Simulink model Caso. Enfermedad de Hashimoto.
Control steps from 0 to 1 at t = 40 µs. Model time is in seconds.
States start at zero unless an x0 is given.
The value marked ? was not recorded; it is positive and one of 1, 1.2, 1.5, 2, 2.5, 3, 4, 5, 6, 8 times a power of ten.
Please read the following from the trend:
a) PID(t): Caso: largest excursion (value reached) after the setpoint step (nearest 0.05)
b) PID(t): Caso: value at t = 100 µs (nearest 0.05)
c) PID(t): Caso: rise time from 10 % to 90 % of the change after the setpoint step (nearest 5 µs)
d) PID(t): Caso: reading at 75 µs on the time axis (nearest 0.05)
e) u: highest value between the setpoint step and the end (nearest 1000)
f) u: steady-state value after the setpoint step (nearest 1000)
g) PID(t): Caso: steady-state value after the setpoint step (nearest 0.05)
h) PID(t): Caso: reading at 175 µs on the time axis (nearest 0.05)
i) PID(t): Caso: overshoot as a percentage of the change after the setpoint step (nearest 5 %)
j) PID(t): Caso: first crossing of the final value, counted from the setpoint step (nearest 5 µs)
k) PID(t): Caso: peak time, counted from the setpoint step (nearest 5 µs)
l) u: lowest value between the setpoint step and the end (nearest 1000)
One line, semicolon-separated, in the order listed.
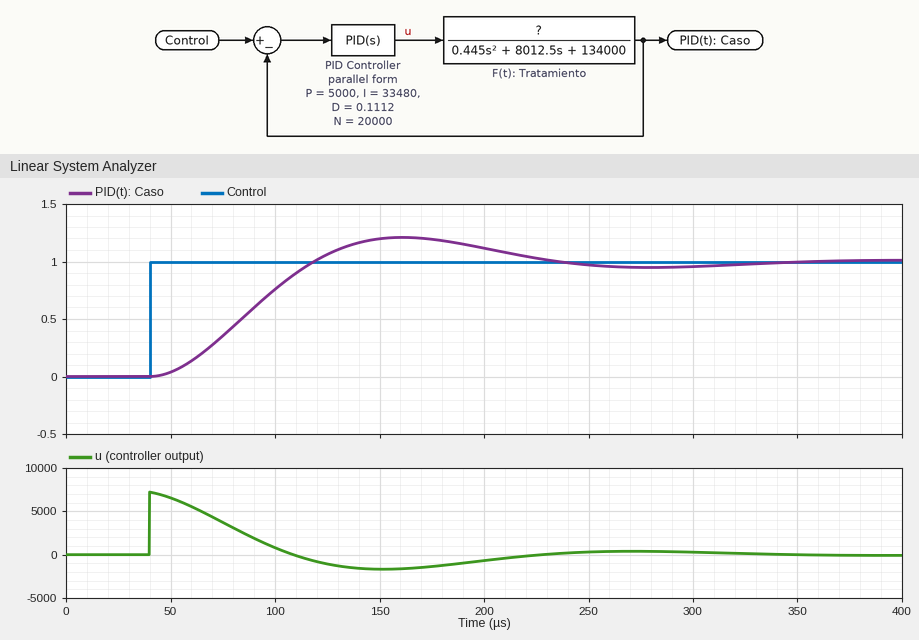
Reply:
1.20; 0.75; 55 µs; 0.35; 7000; 0; 1.00; 1.20; 20 %; 80 µs; 120 µs; -2000
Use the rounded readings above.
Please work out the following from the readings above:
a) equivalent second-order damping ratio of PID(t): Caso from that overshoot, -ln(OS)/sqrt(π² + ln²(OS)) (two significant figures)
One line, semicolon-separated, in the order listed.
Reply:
0.46
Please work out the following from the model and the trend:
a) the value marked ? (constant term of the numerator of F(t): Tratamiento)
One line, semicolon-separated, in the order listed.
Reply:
50000
